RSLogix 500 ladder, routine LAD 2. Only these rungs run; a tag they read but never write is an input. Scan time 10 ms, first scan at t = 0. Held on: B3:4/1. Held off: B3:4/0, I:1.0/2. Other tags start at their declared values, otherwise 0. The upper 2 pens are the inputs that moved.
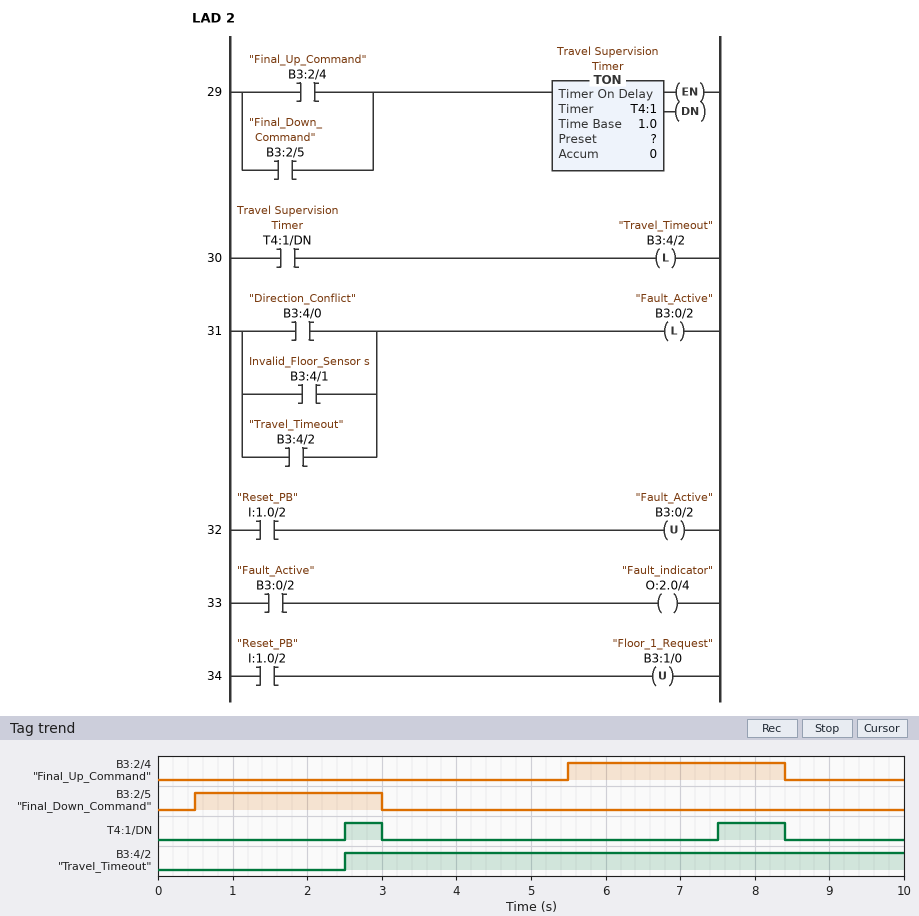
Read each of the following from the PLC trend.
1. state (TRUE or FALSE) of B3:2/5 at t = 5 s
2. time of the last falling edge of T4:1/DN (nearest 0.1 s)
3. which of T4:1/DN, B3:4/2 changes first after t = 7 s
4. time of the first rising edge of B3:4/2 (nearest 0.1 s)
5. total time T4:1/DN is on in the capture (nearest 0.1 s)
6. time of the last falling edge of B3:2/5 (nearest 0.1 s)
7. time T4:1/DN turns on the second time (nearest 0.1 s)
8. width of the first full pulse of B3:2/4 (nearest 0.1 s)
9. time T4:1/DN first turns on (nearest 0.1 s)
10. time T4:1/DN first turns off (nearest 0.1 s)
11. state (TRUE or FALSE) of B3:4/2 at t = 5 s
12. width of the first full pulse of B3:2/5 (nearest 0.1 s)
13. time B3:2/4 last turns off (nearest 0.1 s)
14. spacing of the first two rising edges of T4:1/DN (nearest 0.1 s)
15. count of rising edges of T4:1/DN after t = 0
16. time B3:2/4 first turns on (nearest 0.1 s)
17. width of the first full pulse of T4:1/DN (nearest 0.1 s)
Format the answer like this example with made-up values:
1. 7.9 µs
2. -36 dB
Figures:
1. FALSE
2. 8.4 s
3. T4:1/DN
4. 2.5 s
5. 1.4 s
6. 3.0 s
7. 7.5 s
8. 2.9 s
9. 2.5 s
10. 3.0 s
11. TRUE
12. 2.5 s
13. 8.4 s
14. 5.0 s
15. 2
16. 5.5 s
17. 0.5 s
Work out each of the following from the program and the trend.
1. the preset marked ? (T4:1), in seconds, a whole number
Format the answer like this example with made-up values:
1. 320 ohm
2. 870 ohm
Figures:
1. 2 s
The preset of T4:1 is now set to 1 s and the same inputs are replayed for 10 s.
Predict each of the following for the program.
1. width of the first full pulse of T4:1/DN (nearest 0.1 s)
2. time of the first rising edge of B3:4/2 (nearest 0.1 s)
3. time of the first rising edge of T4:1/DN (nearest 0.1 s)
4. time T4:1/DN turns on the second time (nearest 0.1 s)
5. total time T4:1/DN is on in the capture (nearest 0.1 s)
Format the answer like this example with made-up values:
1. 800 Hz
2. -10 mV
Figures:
1. 1.5 s
2. 1.5 s
3. 1.5 s
4. 6.5 s
5. 3.4 s
